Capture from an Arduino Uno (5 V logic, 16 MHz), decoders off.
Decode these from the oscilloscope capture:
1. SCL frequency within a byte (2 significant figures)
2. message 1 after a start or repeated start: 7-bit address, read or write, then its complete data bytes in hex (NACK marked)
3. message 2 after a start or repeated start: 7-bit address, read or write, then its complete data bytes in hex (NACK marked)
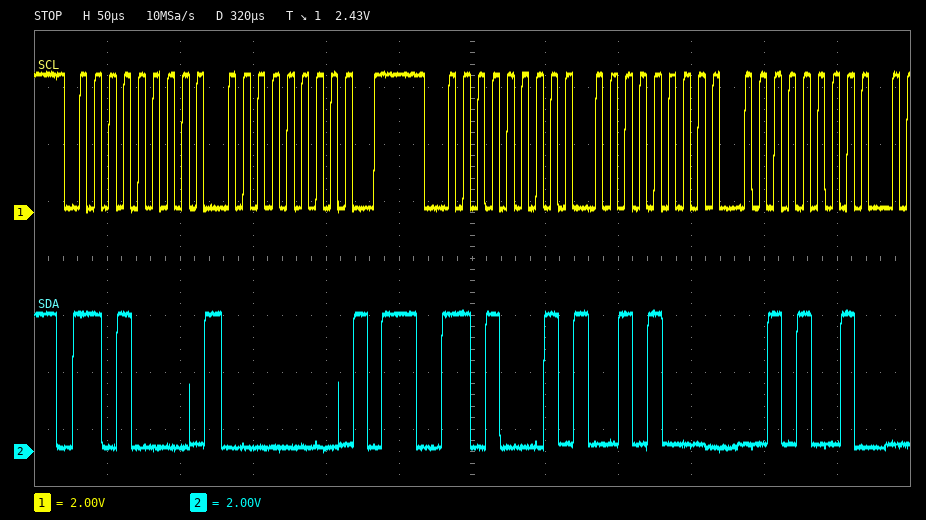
100 kHz
0x68 write: 00
0x68 read: 28 29
